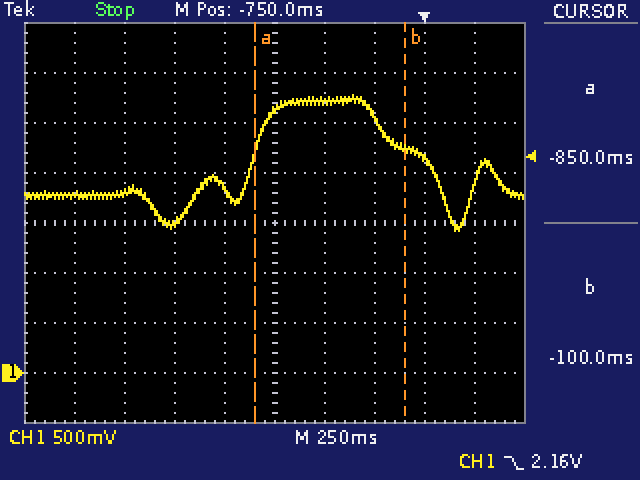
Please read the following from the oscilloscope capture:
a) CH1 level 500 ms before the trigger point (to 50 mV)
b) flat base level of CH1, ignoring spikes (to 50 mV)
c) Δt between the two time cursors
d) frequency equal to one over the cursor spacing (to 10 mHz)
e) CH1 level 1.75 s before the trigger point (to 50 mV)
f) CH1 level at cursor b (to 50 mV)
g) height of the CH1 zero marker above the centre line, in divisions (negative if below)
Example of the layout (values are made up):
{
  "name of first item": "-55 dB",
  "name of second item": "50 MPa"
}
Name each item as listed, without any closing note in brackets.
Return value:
{
  "CH1 level 500 ms before the trigger point": "2.70 V",
  "flat base level of CH1, ignoring spikes": "1.80 V",
  "Δt between the two time cursors": "750 ms",
  "frequency equal to one over the cursor spacing": "1.33 Hz",
  "CH1 level 1.75 s before the trigger point": "1.80 V",
  "CH1 level at cursor b": "2.25 V",
  "height of the CH1 zero marker above the centre line, in divisions": "-3.0 div"
}
